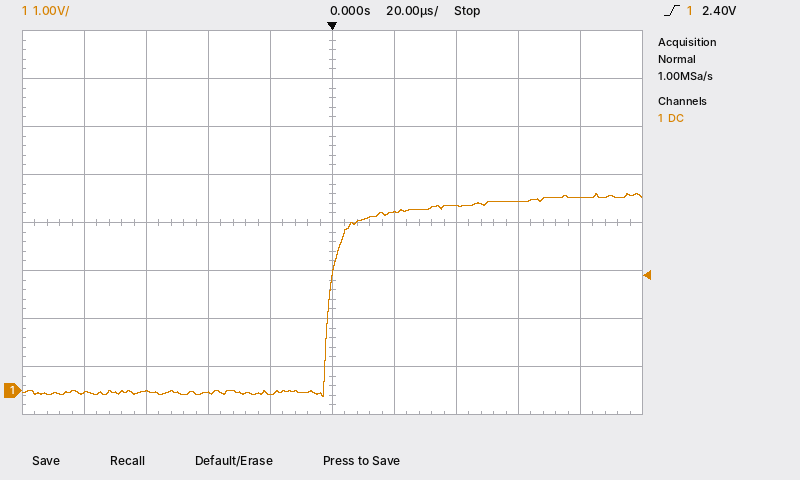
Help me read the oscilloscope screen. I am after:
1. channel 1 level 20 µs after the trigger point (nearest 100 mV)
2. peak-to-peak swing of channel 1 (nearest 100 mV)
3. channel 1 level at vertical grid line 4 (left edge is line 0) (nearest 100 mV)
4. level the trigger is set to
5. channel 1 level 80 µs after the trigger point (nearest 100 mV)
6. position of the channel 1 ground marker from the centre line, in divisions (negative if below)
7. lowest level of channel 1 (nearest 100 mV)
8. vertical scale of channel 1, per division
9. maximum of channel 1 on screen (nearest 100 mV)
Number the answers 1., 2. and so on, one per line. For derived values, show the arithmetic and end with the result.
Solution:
1. 3.7 V
2. 4.1 V − (-100 mV) = 4.2 V
3. -100 mV
4. 2.40 V
5. 4.0 V
6. -3.5 div
7. -100 mV
8. 1 V
9. 4.1 V
